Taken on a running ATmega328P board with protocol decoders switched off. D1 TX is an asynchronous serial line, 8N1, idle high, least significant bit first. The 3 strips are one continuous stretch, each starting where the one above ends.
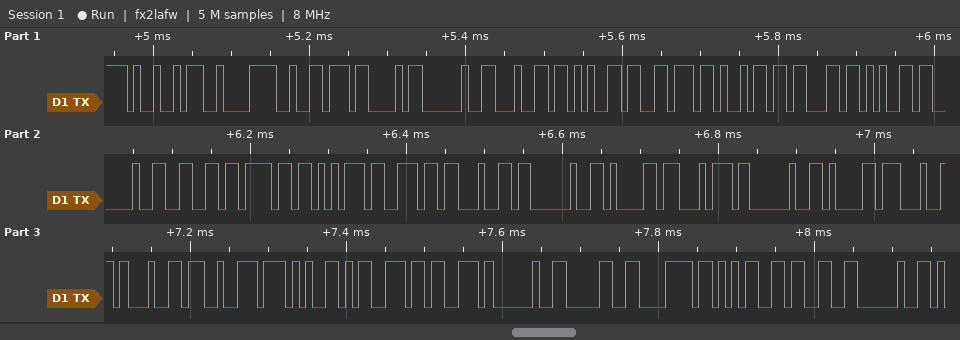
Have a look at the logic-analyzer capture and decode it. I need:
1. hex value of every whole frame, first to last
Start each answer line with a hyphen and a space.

- 49 C2 B2 43 20 64 65 76 69 63 65 20 66 6F 75 6E 64 20 61 74 20 61 64 64 72 65 73 73 20 30 78 35 33 20
